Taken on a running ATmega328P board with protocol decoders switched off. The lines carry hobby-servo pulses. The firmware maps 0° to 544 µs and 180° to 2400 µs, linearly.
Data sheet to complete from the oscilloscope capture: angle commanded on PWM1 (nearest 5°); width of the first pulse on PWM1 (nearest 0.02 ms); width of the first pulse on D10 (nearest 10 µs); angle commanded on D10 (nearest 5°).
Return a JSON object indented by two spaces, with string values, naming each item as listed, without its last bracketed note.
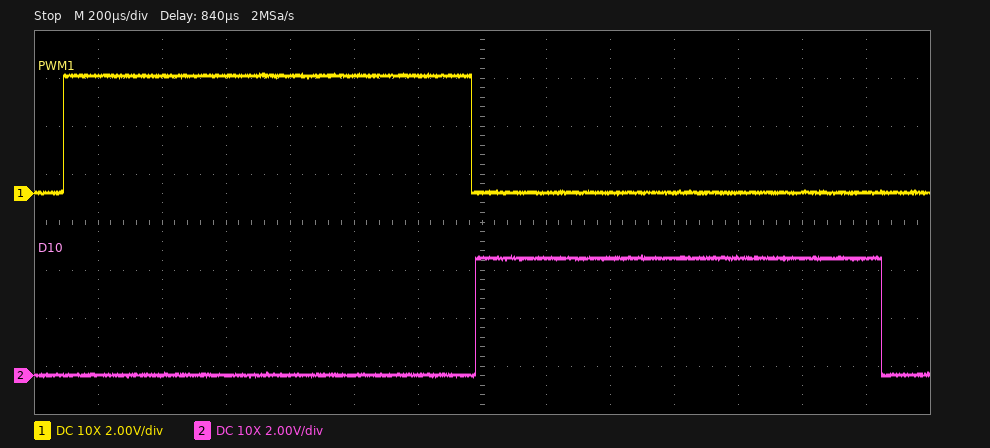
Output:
{
  "angle commanded on PWM1": "70°",
  "width of the first pulse on PWM1": "1.28 ms",
  "width of the first pulse on D10": "1270 µs",
  "angle commanded on D10": "70°"
}
